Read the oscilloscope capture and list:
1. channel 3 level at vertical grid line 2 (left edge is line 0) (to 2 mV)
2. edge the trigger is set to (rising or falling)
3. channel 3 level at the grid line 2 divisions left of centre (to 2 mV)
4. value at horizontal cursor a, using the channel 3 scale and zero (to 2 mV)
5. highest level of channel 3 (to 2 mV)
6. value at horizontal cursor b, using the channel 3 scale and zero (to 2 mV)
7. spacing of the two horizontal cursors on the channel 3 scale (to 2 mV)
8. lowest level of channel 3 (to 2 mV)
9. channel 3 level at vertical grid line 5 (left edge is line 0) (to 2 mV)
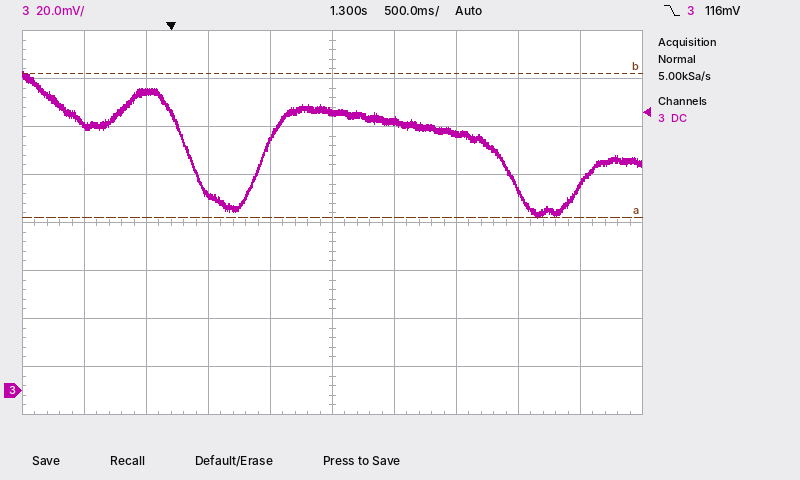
124 mV
falling
82 mV
72 mV
132 mV
132 mV
60 mV
72 mV
116 mV
